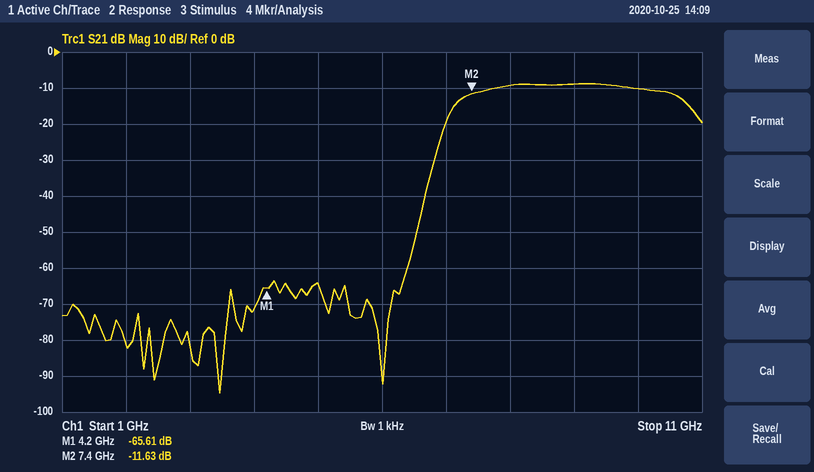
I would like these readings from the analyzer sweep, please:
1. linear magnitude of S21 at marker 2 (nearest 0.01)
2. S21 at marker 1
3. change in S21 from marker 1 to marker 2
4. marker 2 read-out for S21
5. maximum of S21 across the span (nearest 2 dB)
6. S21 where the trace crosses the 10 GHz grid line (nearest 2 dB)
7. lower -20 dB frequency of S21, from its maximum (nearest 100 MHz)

0.26
-65.61 dB
53.98 dB
-11.63 dB
-8 dB
-10 dB
6.8 GHz
